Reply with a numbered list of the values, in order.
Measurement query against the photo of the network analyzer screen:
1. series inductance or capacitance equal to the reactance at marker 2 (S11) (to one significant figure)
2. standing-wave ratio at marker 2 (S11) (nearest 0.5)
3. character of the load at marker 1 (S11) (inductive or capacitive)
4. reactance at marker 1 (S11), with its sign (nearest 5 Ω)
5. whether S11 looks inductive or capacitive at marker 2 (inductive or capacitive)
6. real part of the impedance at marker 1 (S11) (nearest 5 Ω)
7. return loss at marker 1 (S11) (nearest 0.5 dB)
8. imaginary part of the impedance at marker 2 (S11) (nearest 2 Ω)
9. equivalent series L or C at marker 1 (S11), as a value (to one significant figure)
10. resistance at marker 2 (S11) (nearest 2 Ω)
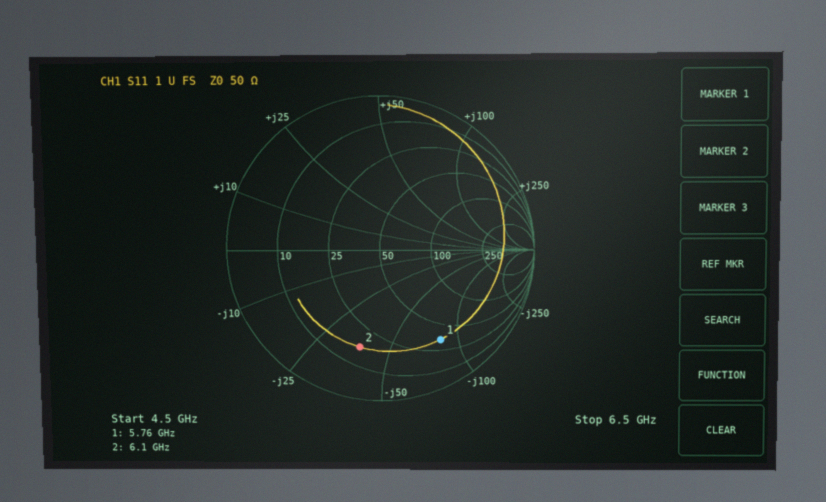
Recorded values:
1. 700 fF
2. 5.0
3. capacitive
4. -80 Ω
5. capacitive
6. 35 Ω
7. 3.0 dB
8. -38 Ω
9. 300 fF
10. 16 Ω
